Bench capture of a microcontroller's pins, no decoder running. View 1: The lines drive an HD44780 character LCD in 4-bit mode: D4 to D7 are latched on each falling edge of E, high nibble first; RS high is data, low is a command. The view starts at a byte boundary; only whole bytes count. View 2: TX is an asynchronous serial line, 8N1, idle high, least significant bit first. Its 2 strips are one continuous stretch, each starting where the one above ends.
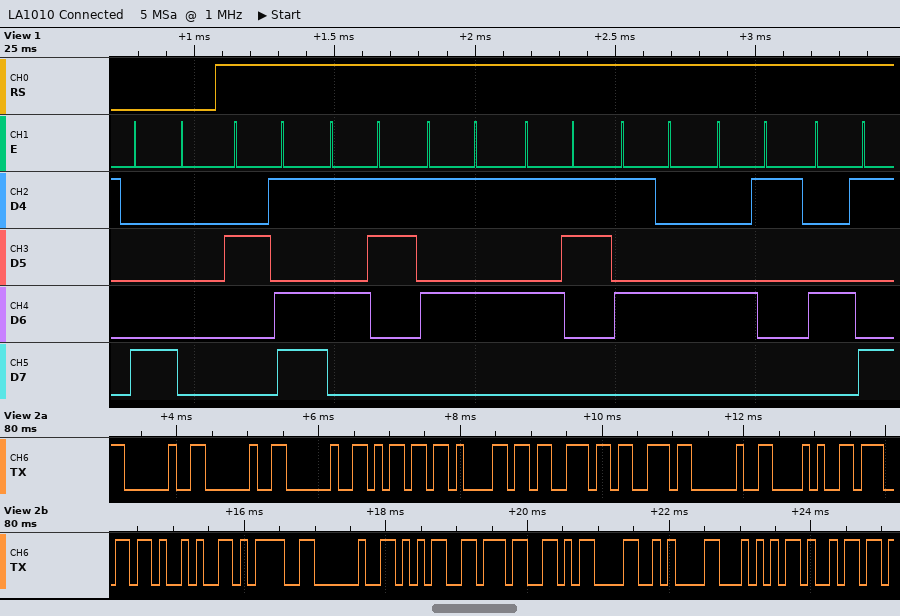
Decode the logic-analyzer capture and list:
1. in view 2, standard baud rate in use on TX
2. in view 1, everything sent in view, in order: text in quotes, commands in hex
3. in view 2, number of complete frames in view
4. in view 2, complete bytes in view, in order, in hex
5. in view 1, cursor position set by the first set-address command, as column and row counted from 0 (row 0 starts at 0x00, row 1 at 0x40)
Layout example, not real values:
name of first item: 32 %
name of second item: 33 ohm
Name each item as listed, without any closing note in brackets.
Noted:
in view 2, standard baud rate in use on TX: 9600 baud
in view 1, everything sent in view, in order: text in quotes, commands in hex: 0x80 "-SUSTAI"
in view 2, number of complete frames in view: 19
in view 2, complete bytes in view, in order, in hex: 0x20 0x20 0x20 0x6D 0x61 0x73 0x73 0x20 0x28 0x67 0x29 0x3D 0x20 0x35 0x37 0x0D 0x0A 0x54 0x69
in view 1, cursor position set by the first set-address command, as column and row counted from 0: column 0, row 0
